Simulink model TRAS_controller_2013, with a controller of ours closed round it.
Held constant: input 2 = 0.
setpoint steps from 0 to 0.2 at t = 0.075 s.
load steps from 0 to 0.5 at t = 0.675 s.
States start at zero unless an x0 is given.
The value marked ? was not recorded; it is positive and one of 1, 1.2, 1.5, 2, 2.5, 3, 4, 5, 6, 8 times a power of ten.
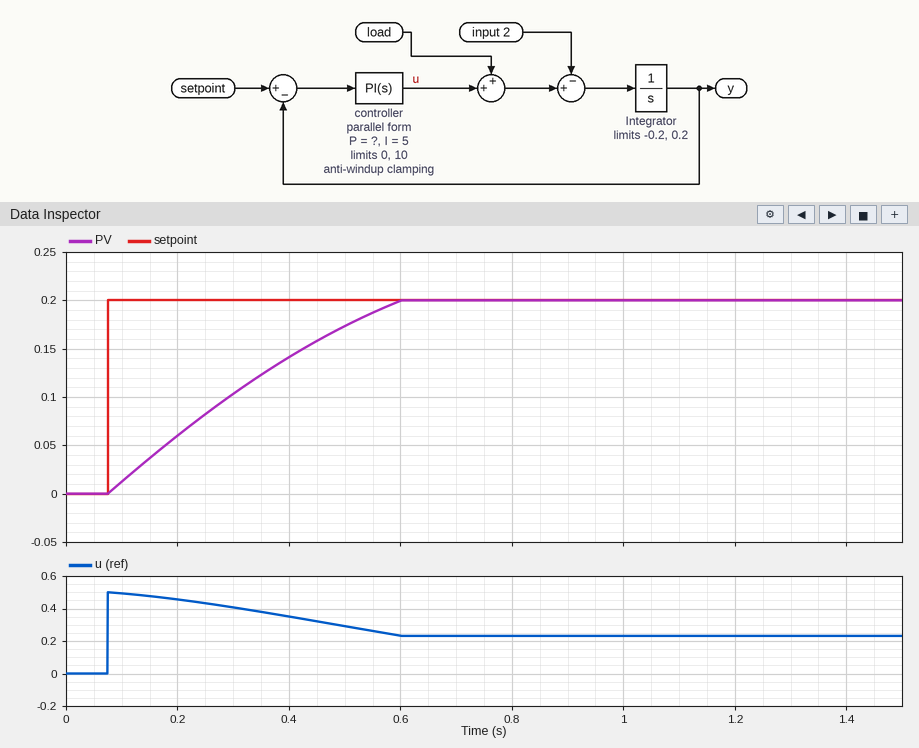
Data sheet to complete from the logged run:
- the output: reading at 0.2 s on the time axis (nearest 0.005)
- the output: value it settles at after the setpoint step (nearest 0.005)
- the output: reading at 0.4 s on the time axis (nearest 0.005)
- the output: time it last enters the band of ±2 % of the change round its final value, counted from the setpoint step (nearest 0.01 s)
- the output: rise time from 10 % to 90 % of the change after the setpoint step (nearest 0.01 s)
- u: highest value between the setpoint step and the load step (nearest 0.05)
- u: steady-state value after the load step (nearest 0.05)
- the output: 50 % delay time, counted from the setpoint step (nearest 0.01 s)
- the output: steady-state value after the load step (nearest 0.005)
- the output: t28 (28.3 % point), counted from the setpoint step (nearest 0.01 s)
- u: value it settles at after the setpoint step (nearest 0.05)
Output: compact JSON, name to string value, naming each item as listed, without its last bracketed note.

{"the output: reading at 0.2 s on the time axis": "0.060", "the output: value it settles at after the setpoint step": "0.200", "the output: reading at 0.4 s on the time axis": "0.140", "the output: time it last enters the band of ±2 % of the change round its final value, counted from the setpoint step": "0.51 s", "the output: rise time from 10 % to 90 % of the change after the setpoint step": "0.41 s", "u: highest value between the setpoint step and the load step": "0.50", "u: steady-state value after the load step": "0.25", "the output: 50 % delay time, counted from the setpoint step": "0.22 s", "the output: steady-state value after the load step": "0.200", "the output: t28 (28.3 % point), counted from the setpoint step": "0.12 s", "u: value it settles at after the setpoint step": "0.25"}
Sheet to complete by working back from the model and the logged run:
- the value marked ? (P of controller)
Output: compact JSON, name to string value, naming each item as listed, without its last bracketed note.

{"the value marked ?": "2.5"}
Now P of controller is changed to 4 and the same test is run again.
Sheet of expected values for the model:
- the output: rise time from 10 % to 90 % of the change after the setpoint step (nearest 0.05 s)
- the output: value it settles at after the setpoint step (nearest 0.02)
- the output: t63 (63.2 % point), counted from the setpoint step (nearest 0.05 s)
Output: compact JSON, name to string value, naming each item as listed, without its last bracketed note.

{"the output: rise time from 10 % to 90 % of the change after the setpoint step": "0.35 s", "the output: value it settles at after the setpoint step": "0.20", "the output: t63 (63.2 % point), counted from the setpoint step": "0.20 s"}
